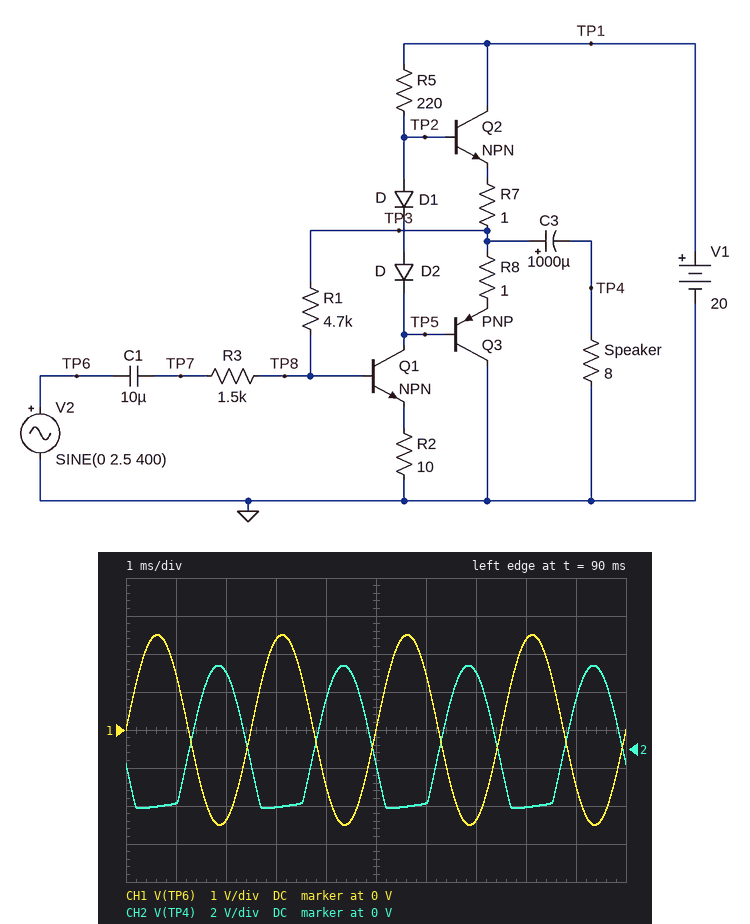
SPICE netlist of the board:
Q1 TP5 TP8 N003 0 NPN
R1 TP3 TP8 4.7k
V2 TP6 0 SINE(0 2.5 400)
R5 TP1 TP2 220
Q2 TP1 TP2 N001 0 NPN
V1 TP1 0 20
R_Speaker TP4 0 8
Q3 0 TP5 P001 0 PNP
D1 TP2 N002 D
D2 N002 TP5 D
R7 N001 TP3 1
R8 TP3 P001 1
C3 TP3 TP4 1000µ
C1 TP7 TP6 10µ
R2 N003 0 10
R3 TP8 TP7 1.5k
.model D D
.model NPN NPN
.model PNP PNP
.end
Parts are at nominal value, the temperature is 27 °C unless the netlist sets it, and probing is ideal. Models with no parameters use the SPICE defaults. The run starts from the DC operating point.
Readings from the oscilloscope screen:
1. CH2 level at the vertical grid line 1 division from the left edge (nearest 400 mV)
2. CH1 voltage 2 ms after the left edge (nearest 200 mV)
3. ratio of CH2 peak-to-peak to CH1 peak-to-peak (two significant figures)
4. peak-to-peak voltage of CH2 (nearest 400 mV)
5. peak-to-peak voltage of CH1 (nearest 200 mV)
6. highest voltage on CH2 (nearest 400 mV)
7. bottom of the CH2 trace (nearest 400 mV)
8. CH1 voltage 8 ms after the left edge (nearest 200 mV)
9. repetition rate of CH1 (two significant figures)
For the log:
-2.8 V
-2.4 V
1.5
7.6 V
5.0 V
4.4 V
-3.2 V
2.4 V
400 Hz
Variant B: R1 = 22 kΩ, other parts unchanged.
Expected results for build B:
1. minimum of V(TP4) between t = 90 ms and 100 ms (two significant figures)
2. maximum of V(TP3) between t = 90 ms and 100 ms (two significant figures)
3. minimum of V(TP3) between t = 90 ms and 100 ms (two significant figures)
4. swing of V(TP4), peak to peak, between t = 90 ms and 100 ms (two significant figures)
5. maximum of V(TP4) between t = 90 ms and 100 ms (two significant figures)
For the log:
-7.7 V
17 V
2.9 V
14 V
6.3 V
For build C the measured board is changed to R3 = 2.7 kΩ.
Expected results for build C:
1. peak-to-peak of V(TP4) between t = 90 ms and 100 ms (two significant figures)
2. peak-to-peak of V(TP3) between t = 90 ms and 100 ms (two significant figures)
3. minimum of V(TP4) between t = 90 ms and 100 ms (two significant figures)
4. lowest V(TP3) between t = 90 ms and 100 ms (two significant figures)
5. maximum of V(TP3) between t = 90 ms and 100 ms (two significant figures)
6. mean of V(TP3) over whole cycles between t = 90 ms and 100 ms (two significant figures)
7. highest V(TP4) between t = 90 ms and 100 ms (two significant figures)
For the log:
5.4 V
5.3 V
-2.5 V
2.2 V
7.6 V
4.7 V
2.8 V
